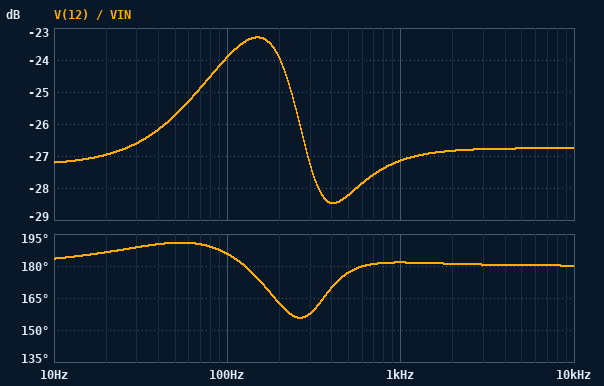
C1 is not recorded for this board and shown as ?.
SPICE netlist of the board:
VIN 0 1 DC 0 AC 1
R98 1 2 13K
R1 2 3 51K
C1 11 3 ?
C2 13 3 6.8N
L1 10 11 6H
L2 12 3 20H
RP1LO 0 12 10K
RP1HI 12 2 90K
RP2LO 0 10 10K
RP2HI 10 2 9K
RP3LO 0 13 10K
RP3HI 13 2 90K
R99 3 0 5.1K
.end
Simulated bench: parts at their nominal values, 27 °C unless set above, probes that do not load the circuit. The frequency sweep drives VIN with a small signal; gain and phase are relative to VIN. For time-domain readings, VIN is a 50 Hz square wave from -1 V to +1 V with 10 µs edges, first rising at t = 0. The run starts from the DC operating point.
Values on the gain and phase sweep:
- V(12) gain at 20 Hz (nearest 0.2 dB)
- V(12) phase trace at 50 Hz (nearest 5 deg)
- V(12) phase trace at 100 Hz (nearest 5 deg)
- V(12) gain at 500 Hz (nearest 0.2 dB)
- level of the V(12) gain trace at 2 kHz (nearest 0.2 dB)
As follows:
-27.0 dB
190 deg
185 deg
-28.2 dB
-26.8 dB
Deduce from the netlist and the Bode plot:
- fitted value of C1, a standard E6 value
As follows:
68 nF
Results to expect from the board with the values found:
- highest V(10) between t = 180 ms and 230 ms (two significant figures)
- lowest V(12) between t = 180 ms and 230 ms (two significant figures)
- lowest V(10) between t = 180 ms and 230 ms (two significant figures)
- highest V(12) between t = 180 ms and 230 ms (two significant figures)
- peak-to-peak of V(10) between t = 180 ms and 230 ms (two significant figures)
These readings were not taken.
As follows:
260 mV
-78 mV
-260 mV
78 mV
520 mV
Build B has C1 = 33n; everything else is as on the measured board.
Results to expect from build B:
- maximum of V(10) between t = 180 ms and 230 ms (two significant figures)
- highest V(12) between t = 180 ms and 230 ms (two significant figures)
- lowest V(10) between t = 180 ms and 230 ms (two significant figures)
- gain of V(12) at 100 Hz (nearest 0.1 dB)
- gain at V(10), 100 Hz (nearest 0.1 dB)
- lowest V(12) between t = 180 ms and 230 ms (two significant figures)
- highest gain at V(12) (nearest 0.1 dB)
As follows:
270 mV
67 mV
-270 mV
-25.5 dB
-12.5 dB
-67 mV
-24.5 dB
